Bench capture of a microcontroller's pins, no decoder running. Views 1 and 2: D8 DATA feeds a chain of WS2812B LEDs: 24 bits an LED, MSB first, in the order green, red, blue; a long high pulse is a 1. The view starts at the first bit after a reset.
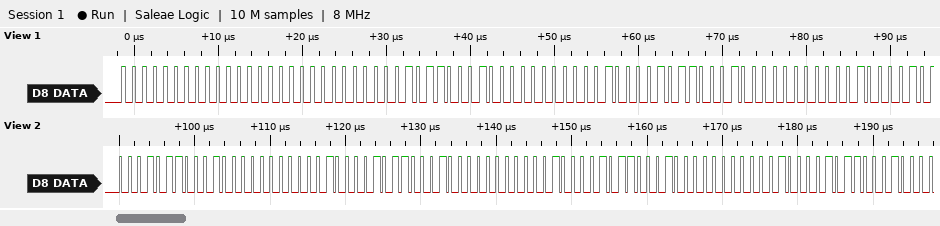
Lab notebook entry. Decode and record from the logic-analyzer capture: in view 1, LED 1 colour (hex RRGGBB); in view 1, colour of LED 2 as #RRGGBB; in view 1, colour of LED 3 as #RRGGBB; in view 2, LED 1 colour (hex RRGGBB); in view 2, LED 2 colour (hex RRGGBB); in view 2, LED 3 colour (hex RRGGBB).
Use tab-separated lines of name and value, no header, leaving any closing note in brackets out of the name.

in view 1, LED 1 colour	#000000
in view 1, colour of LED 2 as #RRGGBB	#201602
in view 1, colour of LED 3 as #RRGGBB	#201602
in view 2, LED 1 colour	#201602
in view 2, LED 2 colour	#201602
in view 2, LED 3 colour	#201602
